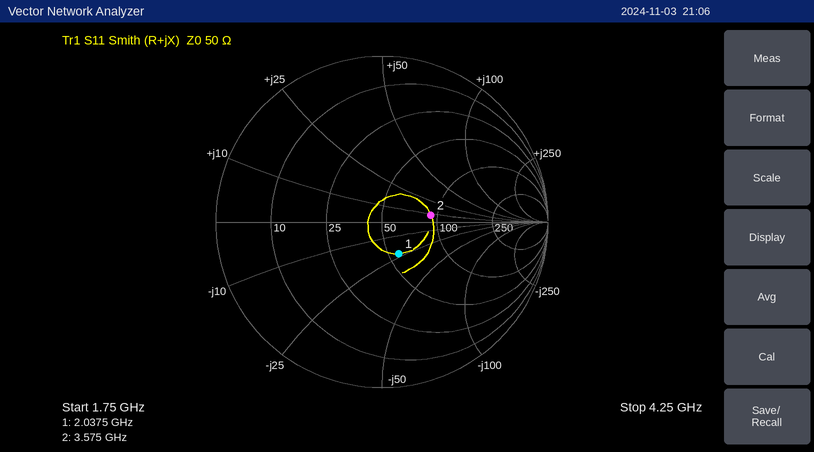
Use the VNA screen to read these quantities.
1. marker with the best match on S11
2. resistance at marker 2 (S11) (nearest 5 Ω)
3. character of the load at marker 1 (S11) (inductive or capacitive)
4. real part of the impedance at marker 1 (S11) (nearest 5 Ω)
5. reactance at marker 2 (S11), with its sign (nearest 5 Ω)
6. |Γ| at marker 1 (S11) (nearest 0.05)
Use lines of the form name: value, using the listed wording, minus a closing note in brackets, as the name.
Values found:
marker with the best match on S11: marker 1
resistance at marker 2 (S11): 90 Ω
character of the load at marker 1 (S11): capacitive
real part of the impedance at marker 1 (S11): 55 Ω
reactance at marker 2 (S11), with its sign: +10 Ω
|Γ| at marker 1 (S11): 0.20
